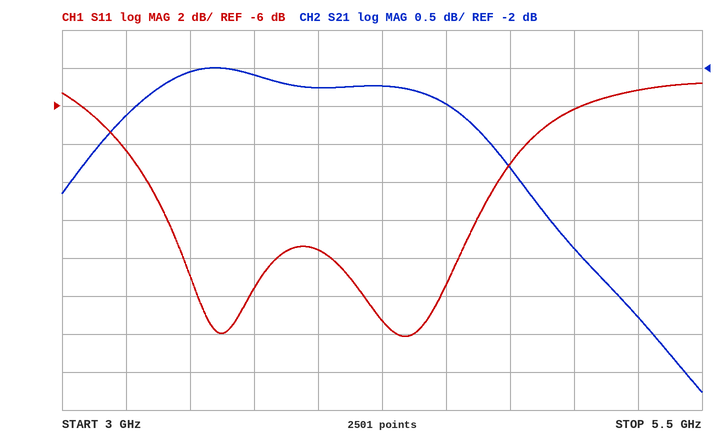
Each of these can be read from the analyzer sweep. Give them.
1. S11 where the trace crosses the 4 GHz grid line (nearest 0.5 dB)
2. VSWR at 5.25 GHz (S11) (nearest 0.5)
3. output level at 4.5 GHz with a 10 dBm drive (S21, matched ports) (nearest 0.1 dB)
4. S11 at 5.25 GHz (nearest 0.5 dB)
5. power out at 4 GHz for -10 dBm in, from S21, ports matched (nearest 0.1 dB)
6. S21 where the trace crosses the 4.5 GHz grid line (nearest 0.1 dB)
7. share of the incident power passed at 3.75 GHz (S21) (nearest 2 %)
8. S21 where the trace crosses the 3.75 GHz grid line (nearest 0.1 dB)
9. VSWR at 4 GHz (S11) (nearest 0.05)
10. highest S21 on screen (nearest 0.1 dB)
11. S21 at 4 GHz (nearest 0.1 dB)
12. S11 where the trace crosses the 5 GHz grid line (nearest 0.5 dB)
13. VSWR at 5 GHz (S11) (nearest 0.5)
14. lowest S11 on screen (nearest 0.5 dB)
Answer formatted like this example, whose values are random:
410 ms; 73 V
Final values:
-13.5 dB; 3.5; 7.5 dBm; -5.0 dB; -12.3 dBm; -2.5 dB; 62 %; -2.1 dB; 1.55; -2.0 dB; -2.3 dB; -6.0 dB; 3.0; -18.0 dB
